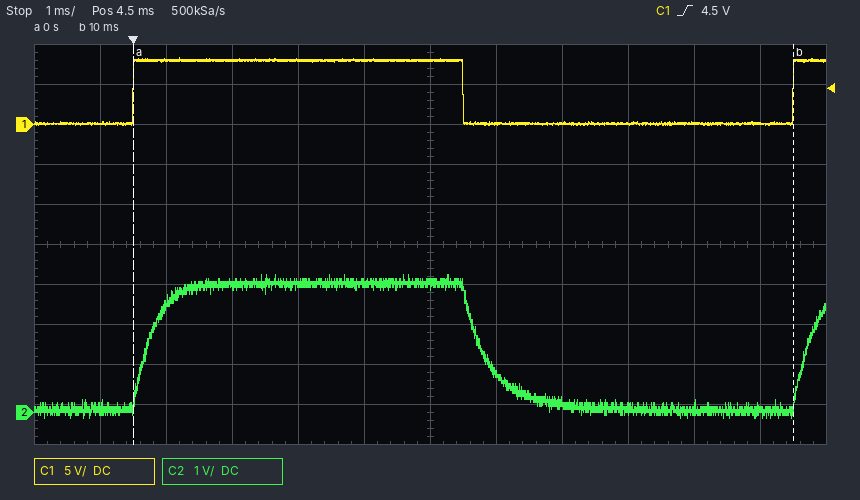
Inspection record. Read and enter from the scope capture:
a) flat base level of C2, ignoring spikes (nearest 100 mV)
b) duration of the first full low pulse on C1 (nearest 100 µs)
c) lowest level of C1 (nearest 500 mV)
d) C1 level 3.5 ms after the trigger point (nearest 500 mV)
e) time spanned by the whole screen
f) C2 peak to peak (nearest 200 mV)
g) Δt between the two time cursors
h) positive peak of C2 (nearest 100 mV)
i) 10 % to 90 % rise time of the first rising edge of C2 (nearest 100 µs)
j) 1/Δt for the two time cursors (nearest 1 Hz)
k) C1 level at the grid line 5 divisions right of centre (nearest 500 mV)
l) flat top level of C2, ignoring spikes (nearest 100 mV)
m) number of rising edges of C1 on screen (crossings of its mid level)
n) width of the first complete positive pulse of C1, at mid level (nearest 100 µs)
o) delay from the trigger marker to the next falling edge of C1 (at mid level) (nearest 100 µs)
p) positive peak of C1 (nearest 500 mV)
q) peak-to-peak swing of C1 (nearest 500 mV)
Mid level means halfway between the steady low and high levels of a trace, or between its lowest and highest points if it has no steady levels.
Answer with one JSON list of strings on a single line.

["100 mV", "5.0 ms", "0.0 V", "8.0 V", "12 ms", "3.6 V", "10.0 ms", "3.4 V", "600 µs", "100 Hz", "0.0 V", "3.2 V", "2", "5.0 ms", "5.0 ms", "8.5 V", "8.5 V"]
